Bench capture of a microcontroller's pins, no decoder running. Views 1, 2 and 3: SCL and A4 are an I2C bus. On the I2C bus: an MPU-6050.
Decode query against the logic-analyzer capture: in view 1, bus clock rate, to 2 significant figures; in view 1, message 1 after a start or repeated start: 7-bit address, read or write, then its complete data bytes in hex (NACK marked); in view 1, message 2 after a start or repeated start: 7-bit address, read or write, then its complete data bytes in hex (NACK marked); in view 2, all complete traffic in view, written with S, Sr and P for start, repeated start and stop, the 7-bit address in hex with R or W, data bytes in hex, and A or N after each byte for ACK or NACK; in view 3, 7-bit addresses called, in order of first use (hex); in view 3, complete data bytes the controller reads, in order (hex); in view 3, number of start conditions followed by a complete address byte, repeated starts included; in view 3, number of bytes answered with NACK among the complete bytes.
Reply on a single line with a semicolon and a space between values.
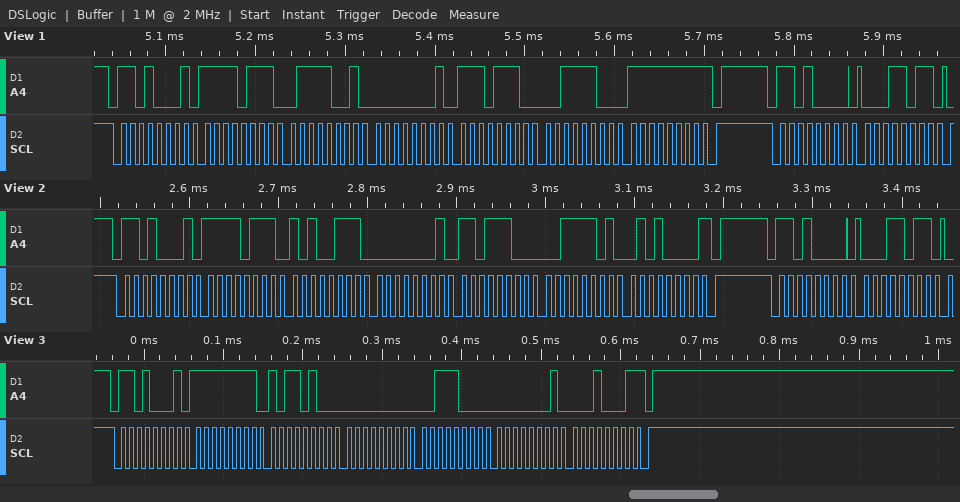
100 kHz; 0x68 read: F7 79 01 EE 3C FF NACK; 0x68 write: 1B; S 68R A F7 A A7 A 01 A DC A 3D A 50 N P S 68W A 1B A; 0x68; FF B4 00 38 01 11; 1; 1
